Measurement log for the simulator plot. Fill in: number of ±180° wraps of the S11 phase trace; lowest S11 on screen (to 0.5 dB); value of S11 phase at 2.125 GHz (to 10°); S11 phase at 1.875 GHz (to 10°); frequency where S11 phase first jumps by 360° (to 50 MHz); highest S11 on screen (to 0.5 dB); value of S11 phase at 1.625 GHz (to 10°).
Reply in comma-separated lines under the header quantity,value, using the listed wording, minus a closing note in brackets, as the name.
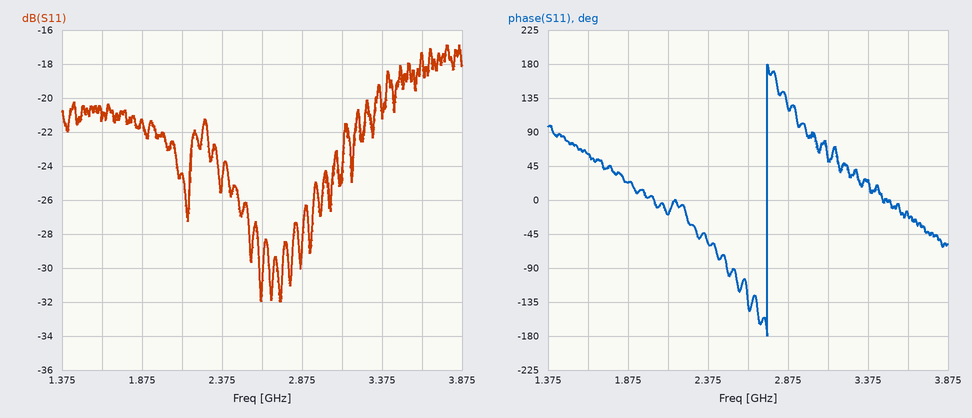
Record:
quantity,value
number of ±180° wraps of the S11 phase trace,1
lowest S11 on screen,-32.0 dB
value of S11 phase at 2.125 GHz,-20°
S11 phase at 1.875 GHz,20°
frequency where S11 phase first jumps by 360°,2.75 GHz
highest S11 on screen,-17.0 dB
value of S11 phase at 1.625 GHz,60°
